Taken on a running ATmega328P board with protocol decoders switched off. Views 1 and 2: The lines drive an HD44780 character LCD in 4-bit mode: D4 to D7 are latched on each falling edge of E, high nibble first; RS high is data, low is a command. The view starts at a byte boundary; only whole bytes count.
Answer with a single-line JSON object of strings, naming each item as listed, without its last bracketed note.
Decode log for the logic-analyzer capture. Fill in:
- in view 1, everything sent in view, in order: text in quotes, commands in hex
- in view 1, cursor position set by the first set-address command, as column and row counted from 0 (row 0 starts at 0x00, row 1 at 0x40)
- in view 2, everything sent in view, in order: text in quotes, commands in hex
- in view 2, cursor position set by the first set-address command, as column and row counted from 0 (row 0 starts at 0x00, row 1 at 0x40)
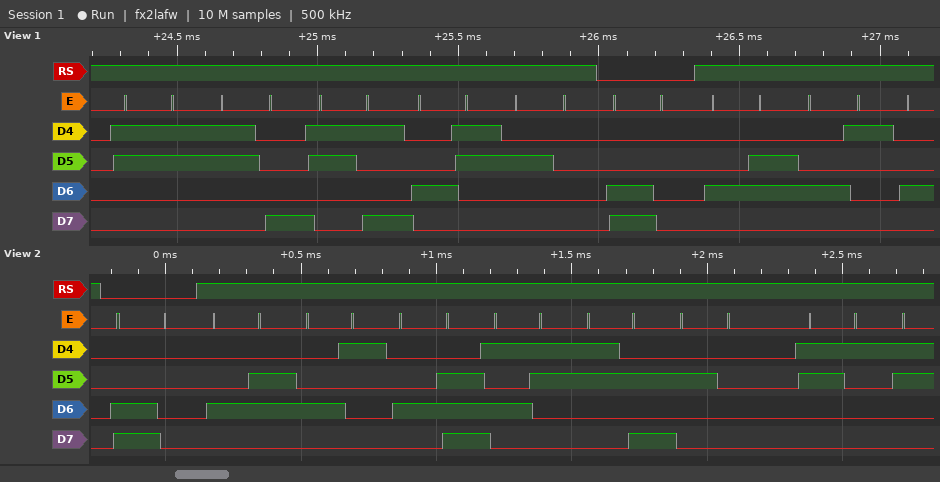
{"in view 1, everything sent in view, in order: text in quotes, commands in hex": "\"389C \" 0xC0 \"FA\"", "in view 1, cursor position set by the first set-address command, as column and row counted from 0": "column 0, row 1", "in view 2, everything sent in view, in order: text in quotes, commands in hex": "0xC0 \"FANS: 1\"", "in view 2, cursor position set by the first set-address command, as column and row counted from 0": "column 0, row 1"}
